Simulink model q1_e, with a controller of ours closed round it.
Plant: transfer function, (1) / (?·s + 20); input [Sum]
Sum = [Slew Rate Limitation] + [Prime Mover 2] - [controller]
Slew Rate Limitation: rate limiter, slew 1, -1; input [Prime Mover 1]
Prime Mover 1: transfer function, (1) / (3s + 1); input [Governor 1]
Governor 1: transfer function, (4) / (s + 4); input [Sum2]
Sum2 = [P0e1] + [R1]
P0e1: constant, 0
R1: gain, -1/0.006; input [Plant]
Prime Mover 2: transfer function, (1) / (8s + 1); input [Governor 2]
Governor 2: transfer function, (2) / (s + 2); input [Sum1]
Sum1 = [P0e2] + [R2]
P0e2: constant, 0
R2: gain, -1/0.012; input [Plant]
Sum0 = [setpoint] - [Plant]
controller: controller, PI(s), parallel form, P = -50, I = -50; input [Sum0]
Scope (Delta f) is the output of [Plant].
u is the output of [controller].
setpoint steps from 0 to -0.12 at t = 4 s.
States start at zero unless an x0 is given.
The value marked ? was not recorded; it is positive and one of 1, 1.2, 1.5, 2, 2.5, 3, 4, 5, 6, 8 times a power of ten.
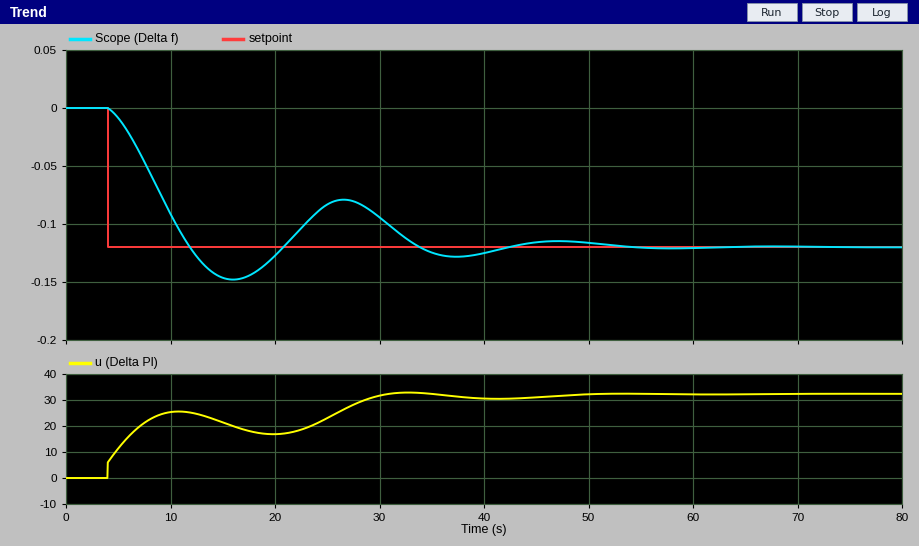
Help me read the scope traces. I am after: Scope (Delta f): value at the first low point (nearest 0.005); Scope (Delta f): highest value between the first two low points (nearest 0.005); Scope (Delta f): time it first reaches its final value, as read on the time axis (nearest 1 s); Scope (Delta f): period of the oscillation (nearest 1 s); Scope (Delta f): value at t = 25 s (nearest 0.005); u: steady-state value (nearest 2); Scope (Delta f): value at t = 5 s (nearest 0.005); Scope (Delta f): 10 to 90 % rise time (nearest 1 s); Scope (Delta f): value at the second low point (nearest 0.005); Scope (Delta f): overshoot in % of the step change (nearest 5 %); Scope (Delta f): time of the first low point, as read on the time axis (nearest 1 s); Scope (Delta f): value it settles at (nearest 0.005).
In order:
-0.150
-0.080
12 s
21 s
-0.085
32
-0.010
6 s
-0.130
25 %
16 s
-0.120
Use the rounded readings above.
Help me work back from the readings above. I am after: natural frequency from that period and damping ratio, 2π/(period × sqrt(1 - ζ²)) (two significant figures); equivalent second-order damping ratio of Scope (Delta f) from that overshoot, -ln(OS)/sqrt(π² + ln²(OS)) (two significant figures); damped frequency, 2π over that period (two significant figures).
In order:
0.33 rad/s
0.40
0.30 rad/s
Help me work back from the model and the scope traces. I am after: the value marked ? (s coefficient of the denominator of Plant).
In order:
1000
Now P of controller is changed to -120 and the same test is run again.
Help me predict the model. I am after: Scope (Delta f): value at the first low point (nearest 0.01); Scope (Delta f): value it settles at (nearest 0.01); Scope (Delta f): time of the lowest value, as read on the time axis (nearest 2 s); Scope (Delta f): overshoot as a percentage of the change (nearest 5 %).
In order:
-0.13
-0.12
14 s
10 %
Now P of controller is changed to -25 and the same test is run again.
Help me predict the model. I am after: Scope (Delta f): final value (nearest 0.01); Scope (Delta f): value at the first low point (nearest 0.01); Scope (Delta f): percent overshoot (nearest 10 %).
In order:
-0.12
-0.16
30 %
